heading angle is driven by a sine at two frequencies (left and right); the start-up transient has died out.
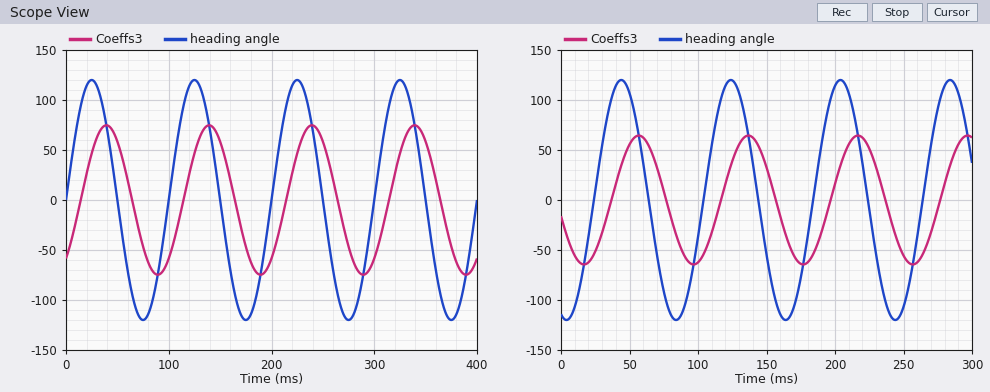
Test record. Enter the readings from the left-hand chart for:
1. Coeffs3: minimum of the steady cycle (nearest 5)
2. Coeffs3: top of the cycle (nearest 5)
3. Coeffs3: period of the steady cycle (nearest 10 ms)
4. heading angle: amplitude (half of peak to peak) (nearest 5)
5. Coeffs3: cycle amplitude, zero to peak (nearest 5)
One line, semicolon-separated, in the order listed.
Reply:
-75; 75; 100 ms; 120; 75
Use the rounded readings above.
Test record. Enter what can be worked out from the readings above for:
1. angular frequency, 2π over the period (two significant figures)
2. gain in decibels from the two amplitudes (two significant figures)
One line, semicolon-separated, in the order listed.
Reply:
0.063 rad/ms; -4.1 dB
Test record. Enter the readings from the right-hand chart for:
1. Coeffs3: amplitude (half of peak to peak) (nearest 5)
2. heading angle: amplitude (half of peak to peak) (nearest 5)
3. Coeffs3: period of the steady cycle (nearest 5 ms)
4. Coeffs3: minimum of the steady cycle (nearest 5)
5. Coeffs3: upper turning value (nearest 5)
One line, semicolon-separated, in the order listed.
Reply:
65; 120; 80 ms; -65; 65
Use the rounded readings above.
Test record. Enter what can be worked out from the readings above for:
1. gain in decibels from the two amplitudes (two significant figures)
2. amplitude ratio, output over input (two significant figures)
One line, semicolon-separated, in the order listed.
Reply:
-5.3 dB; 0.54
